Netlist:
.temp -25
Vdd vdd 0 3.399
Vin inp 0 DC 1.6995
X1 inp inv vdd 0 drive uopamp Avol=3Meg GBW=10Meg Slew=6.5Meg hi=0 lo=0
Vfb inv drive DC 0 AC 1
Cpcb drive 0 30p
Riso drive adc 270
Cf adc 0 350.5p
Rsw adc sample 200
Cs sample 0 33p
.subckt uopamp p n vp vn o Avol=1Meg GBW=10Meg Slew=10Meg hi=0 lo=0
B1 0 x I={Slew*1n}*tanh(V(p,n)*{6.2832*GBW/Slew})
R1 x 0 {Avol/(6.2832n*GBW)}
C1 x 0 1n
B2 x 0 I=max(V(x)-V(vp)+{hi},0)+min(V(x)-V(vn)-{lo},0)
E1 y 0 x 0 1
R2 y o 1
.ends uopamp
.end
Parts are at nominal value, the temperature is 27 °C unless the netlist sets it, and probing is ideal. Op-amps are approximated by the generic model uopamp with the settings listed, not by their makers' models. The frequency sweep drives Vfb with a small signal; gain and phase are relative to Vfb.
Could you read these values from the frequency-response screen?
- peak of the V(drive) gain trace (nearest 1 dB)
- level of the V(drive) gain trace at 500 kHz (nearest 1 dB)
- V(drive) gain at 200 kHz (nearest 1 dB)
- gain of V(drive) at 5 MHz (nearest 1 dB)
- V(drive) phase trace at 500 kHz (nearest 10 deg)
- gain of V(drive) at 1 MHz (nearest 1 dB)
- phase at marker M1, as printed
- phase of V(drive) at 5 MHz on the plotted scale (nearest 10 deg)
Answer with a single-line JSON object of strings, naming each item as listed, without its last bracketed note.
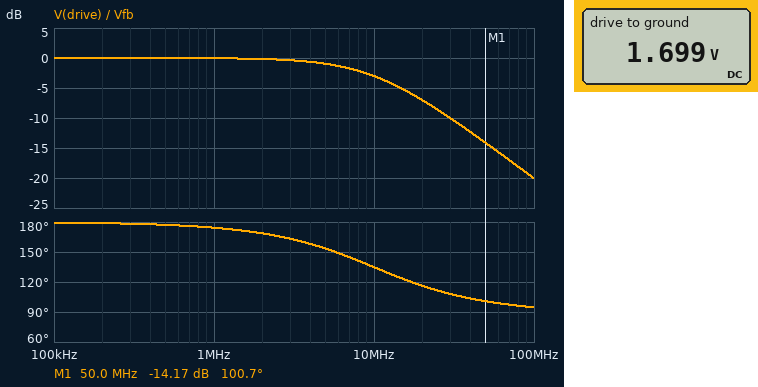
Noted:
{"peak of the V(drive) gain trace": "0 dB", "level of the V(drive) gain trace at 500 kHz": "0 dB", "V(drive) gain at 200 kHz": "0 dB", "gain of V(drive) at 5 MHz": "-1 dB", "V(drive) phase trace at 500 kHz": "180 deg", "gain of V(drive) at 1 MHz": "0 dB", "phase at marker M1, as printed": "100.7 deg", "phase of V(drive) at 5 MHz on the plotted scale": "150 deg"}
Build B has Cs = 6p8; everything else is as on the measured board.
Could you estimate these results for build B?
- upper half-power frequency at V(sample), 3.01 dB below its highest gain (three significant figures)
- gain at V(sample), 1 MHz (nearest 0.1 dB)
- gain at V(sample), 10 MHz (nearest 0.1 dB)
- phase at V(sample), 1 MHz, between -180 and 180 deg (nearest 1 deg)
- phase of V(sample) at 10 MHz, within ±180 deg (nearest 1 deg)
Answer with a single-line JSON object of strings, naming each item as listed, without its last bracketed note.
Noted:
{"upper half-power frequency at V(sample), 3.01 dB below its highest gain": "1.61 MHz", "gain at V(sample), 1 MHz": "-1.4 dB", "gain at V(sample), 10 MHz": "-18.8 dB", "phase at V(sample), 1 MHz, between -180 and 180 deg": "143 deg", "phase of V(sample) at 10 MHz, within ±180 deg": "49 deg"}
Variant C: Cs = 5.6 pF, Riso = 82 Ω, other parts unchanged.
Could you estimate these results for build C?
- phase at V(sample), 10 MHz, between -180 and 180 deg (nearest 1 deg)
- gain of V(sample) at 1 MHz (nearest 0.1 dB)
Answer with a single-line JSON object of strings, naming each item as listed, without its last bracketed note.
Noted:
{"phase at V(sample), 10 MHz, between -180 and 180 deg": "69 deg", "gain of V(sample) at 1 MHz": "-0.2 dB"}
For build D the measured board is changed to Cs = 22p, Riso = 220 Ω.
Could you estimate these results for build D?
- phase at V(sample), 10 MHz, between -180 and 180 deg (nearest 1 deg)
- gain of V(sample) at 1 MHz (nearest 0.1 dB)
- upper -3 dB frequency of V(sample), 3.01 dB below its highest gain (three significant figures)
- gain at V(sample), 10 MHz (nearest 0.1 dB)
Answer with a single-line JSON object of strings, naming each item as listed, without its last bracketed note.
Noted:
{"phase at V(sample), 10 MHz, between -180 and 180 deg": "41 deg", "gain of V(sample) at 1 MHz": "-1.1 dB", "upper -3 dB frequency of V(sample), 3.01 dB below its highest gain": "1.87 MHz", "gain at V(sample), 10 MHz": "-17.7 dB"}
